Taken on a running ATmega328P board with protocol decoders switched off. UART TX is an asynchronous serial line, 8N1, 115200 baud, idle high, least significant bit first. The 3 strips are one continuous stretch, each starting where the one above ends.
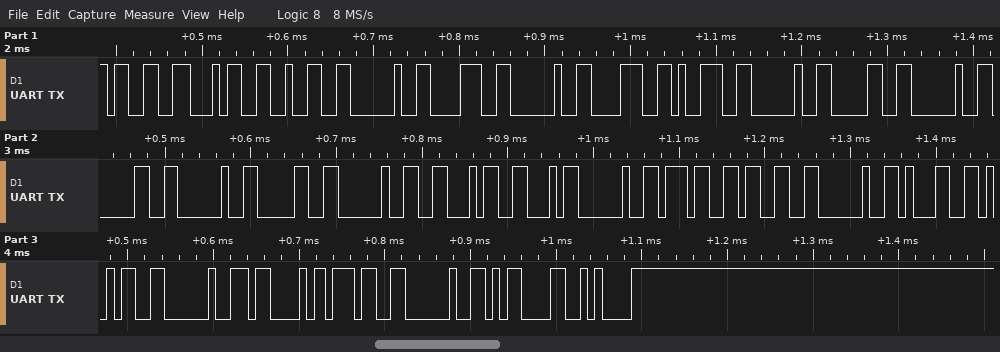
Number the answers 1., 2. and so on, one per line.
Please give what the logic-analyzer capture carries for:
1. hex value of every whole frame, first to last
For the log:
1. 33 34 32 20 38 20 38 39 20 30 20 30 20 30 20 46 46 20 37 33 20 31 35 20 43 37 20 0D 0A
